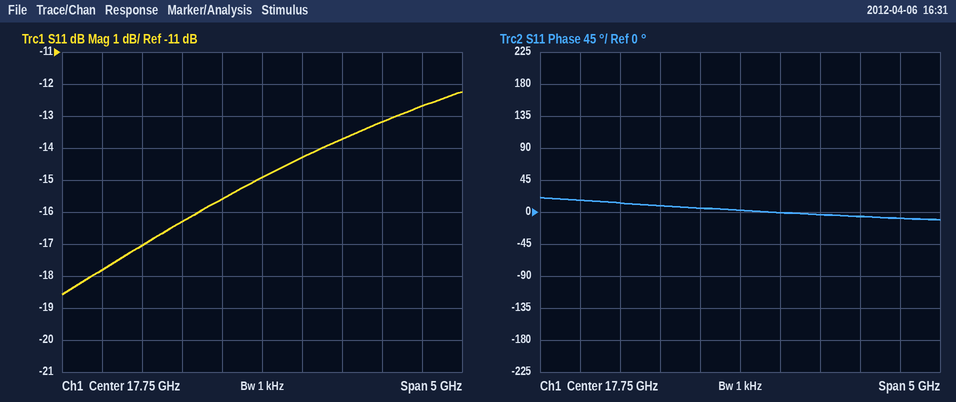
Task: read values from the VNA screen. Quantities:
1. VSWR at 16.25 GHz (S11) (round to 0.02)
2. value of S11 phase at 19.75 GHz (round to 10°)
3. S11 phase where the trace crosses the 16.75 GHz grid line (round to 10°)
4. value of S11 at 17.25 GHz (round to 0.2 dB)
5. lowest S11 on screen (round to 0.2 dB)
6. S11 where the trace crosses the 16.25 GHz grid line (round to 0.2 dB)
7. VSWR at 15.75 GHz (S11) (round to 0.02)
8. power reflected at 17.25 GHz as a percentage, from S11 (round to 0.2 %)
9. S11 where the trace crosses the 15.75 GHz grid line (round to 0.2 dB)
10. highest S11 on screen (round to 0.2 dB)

1.32
-10°
10°
-15.6 dB
-18.6 dB
-17.0 dB
1.30
2.8 %
-17.8 dB
-12.2 dB
